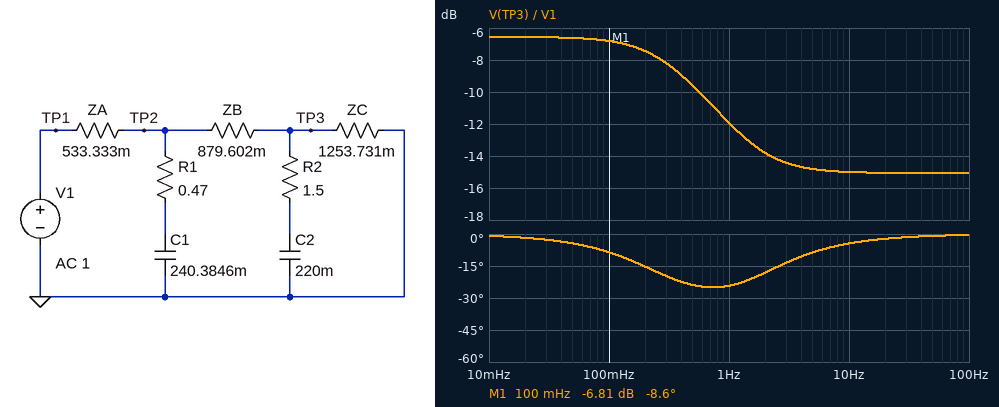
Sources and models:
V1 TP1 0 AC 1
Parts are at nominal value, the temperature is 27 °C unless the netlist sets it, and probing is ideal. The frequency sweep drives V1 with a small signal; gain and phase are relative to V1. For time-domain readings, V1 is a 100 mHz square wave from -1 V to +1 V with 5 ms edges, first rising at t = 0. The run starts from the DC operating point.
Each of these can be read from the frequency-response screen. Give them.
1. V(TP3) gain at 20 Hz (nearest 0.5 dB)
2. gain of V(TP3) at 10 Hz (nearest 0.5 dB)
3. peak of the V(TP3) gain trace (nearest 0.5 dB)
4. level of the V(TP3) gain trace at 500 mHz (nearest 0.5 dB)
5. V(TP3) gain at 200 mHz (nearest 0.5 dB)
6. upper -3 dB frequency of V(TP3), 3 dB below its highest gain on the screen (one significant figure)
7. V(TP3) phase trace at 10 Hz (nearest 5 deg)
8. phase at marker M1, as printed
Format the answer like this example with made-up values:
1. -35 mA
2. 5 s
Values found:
1. -15.0 dB
2. -15.0 dB
3. -6.5 dB
4. -9.5 dB
5. -7.5 dB
6. 500 mHz
7. -5 deg
8. -8.6 deg
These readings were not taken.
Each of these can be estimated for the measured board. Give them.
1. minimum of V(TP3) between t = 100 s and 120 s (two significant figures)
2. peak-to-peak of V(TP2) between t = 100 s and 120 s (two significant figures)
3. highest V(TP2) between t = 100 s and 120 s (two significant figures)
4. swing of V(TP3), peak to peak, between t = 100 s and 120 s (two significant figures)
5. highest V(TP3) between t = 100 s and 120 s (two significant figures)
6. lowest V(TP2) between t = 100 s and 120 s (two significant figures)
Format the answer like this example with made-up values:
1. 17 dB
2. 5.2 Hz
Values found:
1. -470 mV
2. 1.6 V
3. 800 mV
4. 940 mV
5. 470 mV
6. -800 mV
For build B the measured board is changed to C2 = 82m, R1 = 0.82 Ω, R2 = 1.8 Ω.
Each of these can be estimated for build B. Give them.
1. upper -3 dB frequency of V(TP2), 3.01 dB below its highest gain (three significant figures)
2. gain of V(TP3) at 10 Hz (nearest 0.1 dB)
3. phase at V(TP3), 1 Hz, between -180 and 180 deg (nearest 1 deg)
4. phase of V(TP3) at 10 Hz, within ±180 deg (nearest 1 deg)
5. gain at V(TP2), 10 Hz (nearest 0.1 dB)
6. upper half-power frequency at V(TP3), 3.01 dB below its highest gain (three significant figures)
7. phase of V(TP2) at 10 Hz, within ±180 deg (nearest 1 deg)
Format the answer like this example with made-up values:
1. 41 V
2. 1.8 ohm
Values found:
1. 1.14 Hz
2. -12.7 dB
3. -19 deg
4. -3 deg
5. -5.9 dB
6. 719 mHz
7. -2 deg
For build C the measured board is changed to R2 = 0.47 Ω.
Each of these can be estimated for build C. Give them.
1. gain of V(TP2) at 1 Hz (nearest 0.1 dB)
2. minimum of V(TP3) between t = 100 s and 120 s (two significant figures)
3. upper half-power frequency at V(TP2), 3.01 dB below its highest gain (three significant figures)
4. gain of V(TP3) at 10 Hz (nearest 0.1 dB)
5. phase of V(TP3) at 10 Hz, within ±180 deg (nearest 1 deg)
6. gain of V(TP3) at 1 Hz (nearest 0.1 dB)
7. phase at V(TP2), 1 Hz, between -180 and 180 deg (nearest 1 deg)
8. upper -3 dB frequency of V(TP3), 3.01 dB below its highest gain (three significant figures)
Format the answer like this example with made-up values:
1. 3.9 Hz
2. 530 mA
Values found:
1. -5.4 dB
2. -470 mV
3. 857 mHz
4. -19.1 dB
5. -8 deg
6. -13.0 dB
7. -20 deg
8. 522 mHz
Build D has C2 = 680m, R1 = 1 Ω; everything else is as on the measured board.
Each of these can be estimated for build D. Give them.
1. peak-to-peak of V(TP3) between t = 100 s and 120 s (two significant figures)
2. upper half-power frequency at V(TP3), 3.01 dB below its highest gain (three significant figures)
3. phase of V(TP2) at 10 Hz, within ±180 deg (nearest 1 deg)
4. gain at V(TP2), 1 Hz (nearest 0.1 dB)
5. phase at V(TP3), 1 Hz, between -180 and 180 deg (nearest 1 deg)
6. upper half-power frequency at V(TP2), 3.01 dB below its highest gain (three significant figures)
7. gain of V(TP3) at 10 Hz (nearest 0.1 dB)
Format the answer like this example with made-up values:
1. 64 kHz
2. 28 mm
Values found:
1. 920 mV
2. 248 mHz
3. -1 deg
4. -4.8 dB
5. -11 deg
6. 1.22 Hz
7. -12.6 dB
